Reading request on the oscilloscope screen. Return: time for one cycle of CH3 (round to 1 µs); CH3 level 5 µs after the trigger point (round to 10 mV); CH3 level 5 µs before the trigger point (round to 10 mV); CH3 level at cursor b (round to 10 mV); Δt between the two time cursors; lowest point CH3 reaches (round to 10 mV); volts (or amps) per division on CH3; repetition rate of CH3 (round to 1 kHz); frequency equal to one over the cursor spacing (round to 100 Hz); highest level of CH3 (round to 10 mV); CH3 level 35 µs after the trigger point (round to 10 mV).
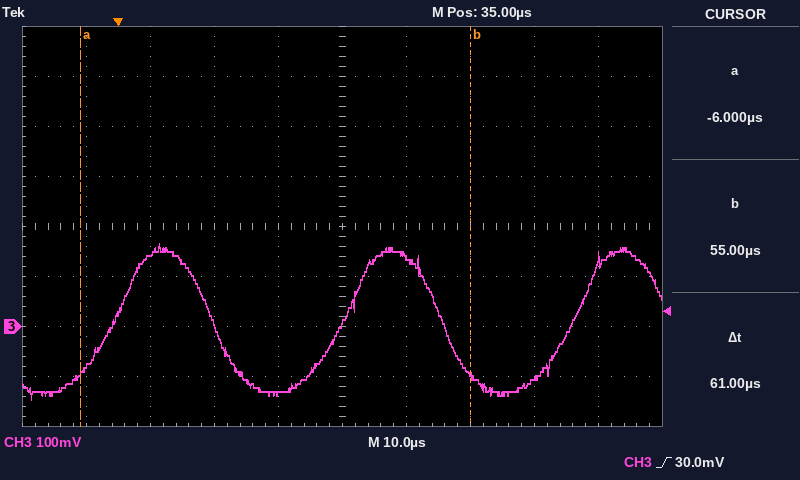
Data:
36 µs
150 mV
-80 mV
-100 mV
61 µs
-150 mV
100 mV
28 kHz
16.4 kHz
170 mV
10 mV
